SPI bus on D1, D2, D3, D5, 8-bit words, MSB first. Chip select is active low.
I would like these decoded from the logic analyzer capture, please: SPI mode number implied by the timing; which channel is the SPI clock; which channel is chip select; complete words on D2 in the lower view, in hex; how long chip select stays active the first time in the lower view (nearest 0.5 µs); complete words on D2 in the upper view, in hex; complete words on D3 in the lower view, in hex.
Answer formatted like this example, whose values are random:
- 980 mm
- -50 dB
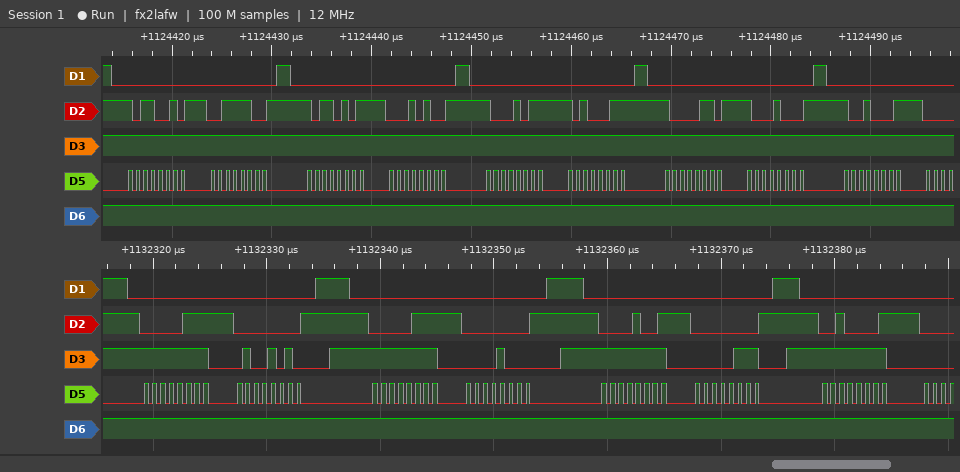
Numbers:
- 0
- D5
- D1
- 07, 00, 07, 00, 09, 00, 21
- 16.5 µs
- B2, 3C, B5, 14, 8B, A3, 86, 88, 91
- FF, 4A, FF, 08, FF, 07, FF
